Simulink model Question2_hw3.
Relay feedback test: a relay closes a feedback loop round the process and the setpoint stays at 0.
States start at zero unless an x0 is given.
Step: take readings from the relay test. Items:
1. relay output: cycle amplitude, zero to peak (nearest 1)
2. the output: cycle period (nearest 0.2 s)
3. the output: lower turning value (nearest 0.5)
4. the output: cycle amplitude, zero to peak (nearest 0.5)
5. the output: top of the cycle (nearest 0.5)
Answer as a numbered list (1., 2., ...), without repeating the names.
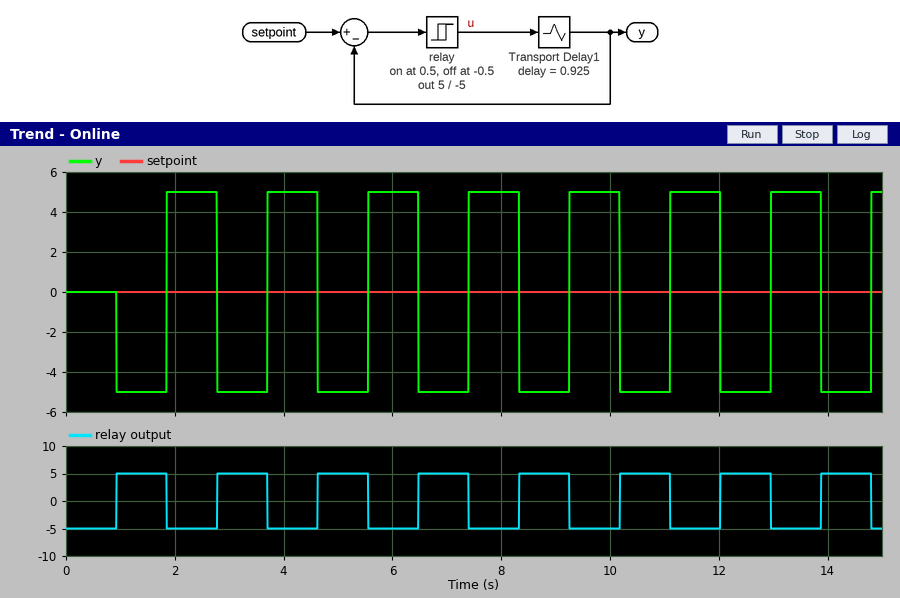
1. 5
2. 1.8 s
3. -5.0
4. 5.0
5. 5.0
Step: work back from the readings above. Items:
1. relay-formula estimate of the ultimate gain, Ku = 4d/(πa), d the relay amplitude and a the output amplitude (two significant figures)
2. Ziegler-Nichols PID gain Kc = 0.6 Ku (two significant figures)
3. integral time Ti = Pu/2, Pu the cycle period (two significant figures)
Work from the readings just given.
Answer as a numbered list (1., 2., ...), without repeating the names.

1. 1.3
2. 0.78
3. 0.90 s
